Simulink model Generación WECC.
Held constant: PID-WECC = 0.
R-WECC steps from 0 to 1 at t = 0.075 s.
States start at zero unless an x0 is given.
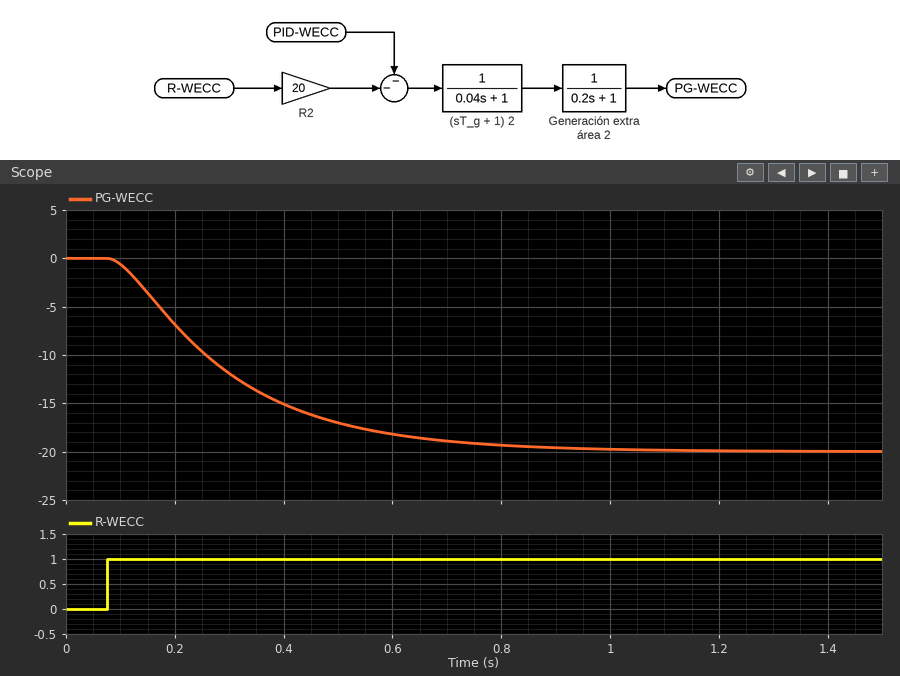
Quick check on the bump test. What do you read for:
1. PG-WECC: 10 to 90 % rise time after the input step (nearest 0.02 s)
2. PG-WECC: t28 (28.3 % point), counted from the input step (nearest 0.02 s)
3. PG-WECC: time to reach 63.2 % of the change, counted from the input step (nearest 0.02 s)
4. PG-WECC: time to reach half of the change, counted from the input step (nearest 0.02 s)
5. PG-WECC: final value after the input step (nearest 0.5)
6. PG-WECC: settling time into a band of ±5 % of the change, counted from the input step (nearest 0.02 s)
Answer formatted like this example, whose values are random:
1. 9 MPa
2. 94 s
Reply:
1. 0.46 s
2. 0.10 s
3. 0.24 s
4. 0.18 s
5. -20.0
6. 0.64 s
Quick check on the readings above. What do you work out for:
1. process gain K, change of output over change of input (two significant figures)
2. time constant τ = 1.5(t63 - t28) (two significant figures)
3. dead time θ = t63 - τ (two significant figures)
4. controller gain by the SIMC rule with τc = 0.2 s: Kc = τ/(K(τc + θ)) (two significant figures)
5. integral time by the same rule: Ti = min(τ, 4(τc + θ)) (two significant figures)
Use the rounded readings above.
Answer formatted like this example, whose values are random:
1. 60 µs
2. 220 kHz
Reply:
1. -20
2. 0.21 s
3. 0.030 s
4. -0.046
5. 0.21 s
